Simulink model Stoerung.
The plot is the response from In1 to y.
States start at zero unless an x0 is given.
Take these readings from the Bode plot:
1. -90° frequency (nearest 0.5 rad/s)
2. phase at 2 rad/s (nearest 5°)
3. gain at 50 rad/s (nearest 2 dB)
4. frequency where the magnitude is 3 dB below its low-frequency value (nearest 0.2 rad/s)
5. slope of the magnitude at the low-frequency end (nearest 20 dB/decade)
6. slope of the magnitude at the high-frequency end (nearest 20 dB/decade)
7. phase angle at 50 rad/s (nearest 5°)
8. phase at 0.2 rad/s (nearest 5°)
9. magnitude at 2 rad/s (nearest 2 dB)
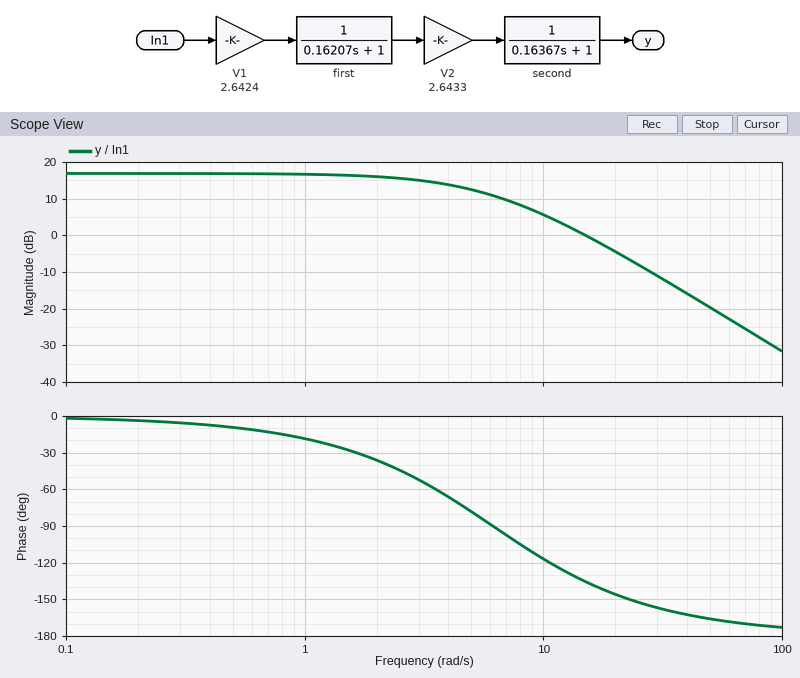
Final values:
6.0 rad/s
-35°
-20 dB
4.0 rad/s
0 dB/decade
-40 dB/decade
-165°
-5°
16 dB
